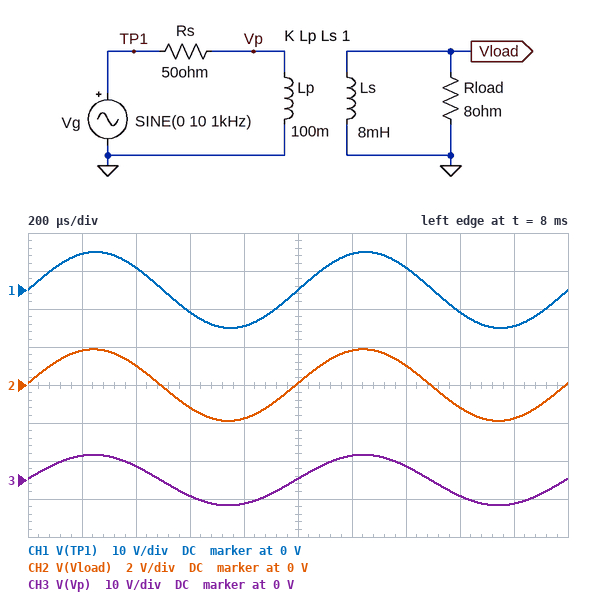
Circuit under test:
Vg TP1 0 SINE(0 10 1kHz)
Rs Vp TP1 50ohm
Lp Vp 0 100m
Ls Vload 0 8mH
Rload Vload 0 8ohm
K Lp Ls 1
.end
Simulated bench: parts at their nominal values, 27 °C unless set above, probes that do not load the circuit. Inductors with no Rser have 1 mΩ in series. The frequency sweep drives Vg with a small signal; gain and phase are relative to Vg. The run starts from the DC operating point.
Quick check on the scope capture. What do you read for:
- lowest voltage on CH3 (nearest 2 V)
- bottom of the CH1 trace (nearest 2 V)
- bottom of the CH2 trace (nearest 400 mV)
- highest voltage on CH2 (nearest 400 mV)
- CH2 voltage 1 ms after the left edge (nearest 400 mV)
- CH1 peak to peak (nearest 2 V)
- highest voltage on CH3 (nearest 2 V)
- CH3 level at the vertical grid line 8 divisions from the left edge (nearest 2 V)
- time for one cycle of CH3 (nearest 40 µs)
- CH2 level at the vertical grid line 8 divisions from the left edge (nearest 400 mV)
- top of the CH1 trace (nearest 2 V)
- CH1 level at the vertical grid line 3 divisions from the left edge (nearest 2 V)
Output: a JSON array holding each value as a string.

["-6 V", "-10 V", "-2.0 V", "2.0 V", "0 V", "20 V", "6 V", "-4 V", "1.00 ms", "-1.2 V", "10 V", "-6 V"]
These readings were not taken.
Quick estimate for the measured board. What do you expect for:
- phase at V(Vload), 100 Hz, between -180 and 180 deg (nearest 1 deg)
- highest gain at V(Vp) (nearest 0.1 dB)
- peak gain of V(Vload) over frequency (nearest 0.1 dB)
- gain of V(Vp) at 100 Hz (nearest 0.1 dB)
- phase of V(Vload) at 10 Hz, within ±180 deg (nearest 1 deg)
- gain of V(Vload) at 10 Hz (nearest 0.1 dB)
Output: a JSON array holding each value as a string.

["28 deg", "-3.5 dB", "-14.5 dB", "-4.6 dB", "79 deg", "-29.1 dB"]
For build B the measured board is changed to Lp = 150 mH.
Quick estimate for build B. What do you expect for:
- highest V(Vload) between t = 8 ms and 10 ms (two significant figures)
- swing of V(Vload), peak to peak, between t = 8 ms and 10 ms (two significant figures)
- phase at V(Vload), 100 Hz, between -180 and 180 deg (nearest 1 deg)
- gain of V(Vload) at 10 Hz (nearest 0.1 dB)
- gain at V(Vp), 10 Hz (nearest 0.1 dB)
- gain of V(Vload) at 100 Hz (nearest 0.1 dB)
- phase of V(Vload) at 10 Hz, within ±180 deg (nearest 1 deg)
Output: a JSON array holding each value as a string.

["1.7 V", "3.5 V", "22 deg", "-27.5 dB", "-14.8 dB", "-15.9 dB", "76 deg"]
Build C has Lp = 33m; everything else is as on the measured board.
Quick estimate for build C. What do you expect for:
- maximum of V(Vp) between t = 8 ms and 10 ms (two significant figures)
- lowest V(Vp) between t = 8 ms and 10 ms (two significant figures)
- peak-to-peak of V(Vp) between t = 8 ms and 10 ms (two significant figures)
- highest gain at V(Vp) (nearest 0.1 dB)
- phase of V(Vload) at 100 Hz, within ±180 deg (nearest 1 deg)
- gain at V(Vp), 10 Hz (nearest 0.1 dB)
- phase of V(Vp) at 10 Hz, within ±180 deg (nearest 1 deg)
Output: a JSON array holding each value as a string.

["4.0 V", "-4.0 V", "7.9 V", "-8.0 dB", "44 deg", "-27.7 dB", "84 deg"]
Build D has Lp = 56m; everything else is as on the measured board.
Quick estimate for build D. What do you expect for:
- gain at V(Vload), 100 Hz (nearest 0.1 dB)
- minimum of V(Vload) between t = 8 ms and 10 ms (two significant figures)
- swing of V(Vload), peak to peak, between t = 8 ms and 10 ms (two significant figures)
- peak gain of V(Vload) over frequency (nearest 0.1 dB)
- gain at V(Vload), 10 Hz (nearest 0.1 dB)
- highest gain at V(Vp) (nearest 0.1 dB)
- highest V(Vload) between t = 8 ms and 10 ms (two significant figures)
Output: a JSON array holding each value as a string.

["-15.9 dB", "-2.0 V", "4.0 V", "-14.0 dB", "-31.6 dB", "-5.5 dB", "2.0 V"]
